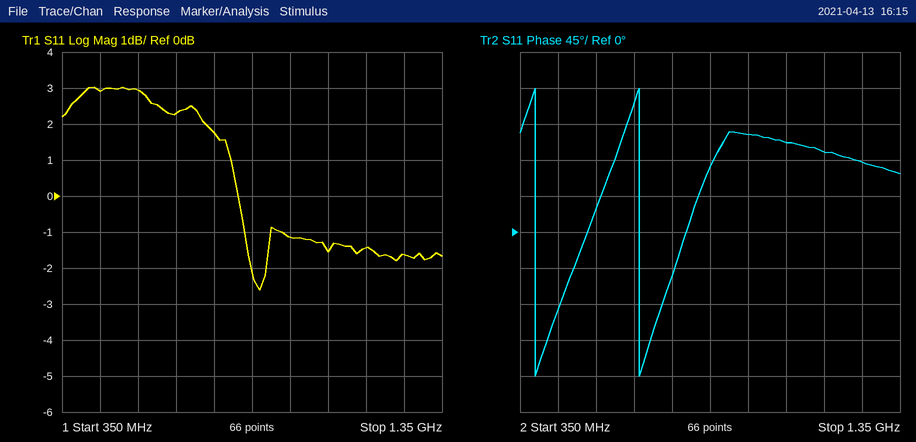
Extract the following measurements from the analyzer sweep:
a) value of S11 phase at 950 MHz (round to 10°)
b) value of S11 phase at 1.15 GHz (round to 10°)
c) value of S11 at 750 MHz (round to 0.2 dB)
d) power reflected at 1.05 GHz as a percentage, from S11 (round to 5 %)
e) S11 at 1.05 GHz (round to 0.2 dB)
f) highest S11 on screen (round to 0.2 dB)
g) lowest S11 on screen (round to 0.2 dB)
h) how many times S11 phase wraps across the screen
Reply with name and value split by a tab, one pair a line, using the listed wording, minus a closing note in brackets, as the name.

value of S11 phase at 950 MHz	120°
value of S11 phase at 1.15 GHz	100°
value of S11 at 750 MHz	1.8 dB
power reflected at 1.05 GHz as a percentage, from S11	70 %
S11 at 1.05 GHz	-1.6 dB
highest S11 on screen	3.0 dB
lowest S11 on screen	-2.6 dB
how many times S11 phase wraps across the screen	2
